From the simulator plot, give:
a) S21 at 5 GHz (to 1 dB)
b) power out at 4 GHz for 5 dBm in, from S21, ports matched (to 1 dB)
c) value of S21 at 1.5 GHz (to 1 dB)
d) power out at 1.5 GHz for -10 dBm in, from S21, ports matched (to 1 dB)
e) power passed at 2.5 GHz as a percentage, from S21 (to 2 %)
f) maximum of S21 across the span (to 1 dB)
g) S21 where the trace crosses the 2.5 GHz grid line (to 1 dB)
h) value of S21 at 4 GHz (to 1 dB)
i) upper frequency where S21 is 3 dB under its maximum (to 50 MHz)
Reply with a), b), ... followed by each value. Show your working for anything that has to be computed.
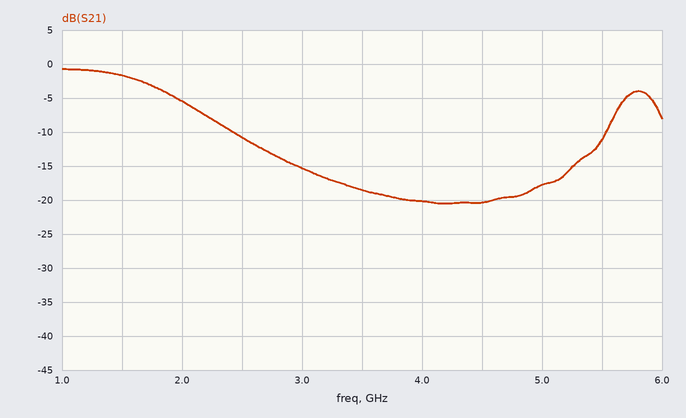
a) -18 dB
b) 5 dBm + (-20 dB) = -15 dBm
c) -2 dB
d) -10 dBm + (-2 dB) = -12 dBm
e) 10^(-11/10) ≈ 8 %
f) -1 dB
g) -11 dB
h) -20 dB
i) 1.80 GHz
